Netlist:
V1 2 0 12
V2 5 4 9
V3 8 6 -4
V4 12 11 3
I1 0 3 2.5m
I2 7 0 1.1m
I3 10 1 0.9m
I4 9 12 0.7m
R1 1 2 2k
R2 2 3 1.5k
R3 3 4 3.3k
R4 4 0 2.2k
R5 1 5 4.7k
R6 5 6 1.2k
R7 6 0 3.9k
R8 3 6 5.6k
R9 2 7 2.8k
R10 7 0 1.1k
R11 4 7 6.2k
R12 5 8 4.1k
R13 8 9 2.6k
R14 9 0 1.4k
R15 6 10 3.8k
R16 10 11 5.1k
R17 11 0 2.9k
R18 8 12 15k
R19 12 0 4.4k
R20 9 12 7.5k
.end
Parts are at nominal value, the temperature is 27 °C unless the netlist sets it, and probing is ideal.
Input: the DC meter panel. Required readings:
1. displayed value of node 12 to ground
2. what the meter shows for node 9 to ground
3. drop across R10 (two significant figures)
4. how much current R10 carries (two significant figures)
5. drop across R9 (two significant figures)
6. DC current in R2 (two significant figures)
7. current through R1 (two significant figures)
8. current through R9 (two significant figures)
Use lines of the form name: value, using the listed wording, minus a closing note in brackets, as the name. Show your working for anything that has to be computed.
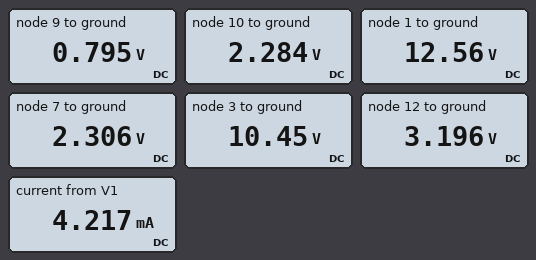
displayed value of node 12 to ground: 3.196 V
what the meter shows for node 9 to ground: 0.795 V
drop across R10: 2.306 V = 2.3 V
how much current R10 carries: (2.306 V) / 1.1 kΩ = 2.1 mA
drop across R9: 12 V - 2.306 V = 9.7 V
DC current in R2: (12 V - 10.45 V) / 1.5 kΩ = 1.0 mA
current through R1: (12.56 V - 12 V) / 2 kΩ = 280 µA
current through R9: (12 V - 2.306 V) / 2.8 kΩ = 3.5 mA
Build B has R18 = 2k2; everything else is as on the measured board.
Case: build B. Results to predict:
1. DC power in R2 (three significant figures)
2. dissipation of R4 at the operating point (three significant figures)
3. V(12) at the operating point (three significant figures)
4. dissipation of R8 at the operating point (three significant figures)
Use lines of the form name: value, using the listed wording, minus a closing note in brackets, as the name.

DC power in R2: 1.62 mW
dissipation of R4 at the operating point: 192 µW
V(12) at the operating point: 3.21 V
dissipation of R8 at the operating point: 1.82 mW
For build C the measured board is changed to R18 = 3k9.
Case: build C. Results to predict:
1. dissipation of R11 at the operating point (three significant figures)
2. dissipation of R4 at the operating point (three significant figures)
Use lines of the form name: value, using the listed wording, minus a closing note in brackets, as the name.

dissipation of R11 at the operating point: 441 µW
dissipation of R4 at the operating point: 193 µW
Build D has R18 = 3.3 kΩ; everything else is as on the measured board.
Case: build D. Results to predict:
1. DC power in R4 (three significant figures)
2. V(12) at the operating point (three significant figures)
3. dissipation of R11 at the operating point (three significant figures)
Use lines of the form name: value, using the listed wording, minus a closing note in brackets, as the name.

DC power in R4: 193 µW
V(12) at the operating point: 3.21 V
dissipation of R11 at the operating point: 441 µW
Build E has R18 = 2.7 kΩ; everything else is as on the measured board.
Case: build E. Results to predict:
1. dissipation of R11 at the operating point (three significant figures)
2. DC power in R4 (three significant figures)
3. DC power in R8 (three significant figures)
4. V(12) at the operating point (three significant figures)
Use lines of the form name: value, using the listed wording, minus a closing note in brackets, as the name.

dissipation of R11 at the operating point: 442 µW
DC power in R4: 192 µW
DC power in R8: 1.82 mW
V(12) at the operating point: 3.21 V
